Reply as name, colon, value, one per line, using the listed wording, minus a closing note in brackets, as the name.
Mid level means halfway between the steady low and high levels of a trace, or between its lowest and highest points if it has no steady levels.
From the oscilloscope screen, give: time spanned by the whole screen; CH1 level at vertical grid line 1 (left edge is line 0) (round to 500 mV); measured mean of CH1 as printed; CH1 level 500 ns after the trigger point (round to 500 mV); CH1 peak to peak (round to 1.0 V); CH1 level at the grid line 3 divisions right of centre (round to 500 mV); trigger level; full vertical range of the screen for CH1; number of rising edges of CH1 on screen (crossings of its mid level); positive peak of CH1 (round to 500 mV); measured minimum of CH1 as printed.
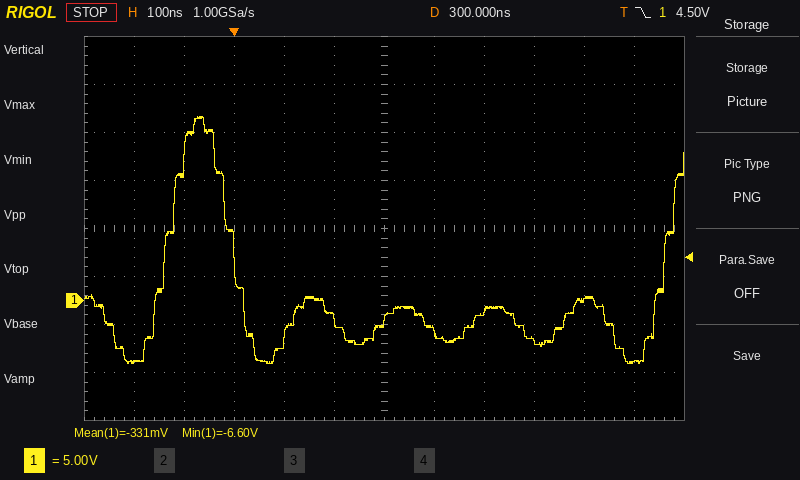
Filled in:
time spanned by the whole screen: 1.2 µs
CH1 level at vertical grid line 1 (left edge is line 0): -6.5 V
measured mean of CH1 as printed: -331 mV
CH1 level 500 ns after the trigger point: -1.0 V
CH1 peak to peak: 26.0 V
CH1 level at the grid line 3 divisions right of centre: -4.0 V
trigger level: 4.50 V
full vertical range of the screen for CH1: 40 V
number of rising edges of CH1 on screen: 2
positive peak of CH1: 19.0 V
measured minimum of CH1 as printed: -6.60 V
